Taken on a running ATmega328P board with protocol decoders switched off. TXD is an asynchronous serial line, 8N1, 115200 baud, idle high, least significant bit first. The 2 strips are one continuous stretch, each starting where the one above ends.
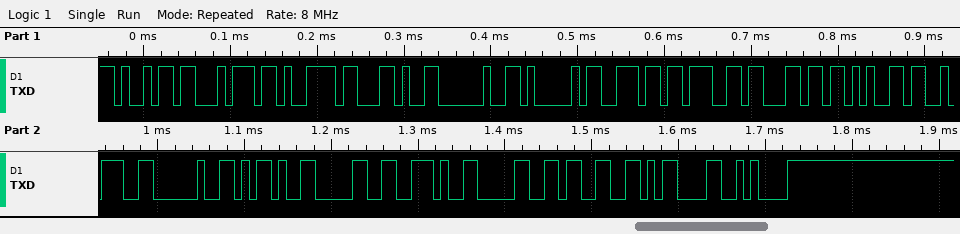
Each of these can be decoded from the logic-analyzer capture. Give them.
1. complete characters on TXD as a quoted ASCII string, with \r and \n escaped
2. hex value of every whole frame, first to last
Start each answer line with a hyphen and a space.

- "ity, Angle: -0.03\r\n"
- 69 74 79 2C 20 41 6E 67 6C 65 3A 20 2D 30 2E 30 33 0D 0A
